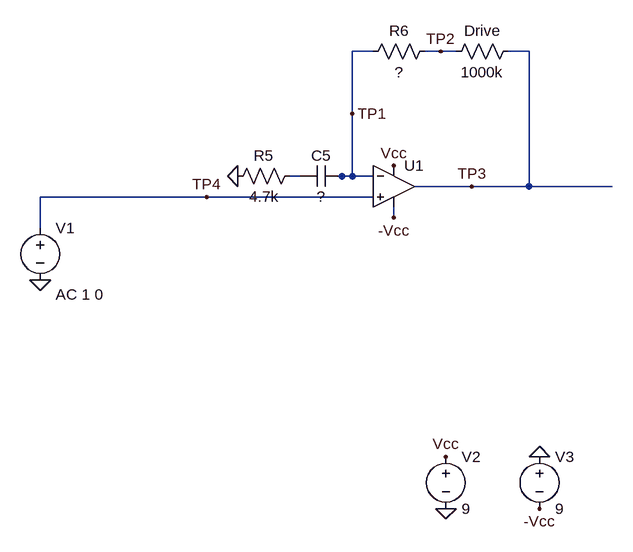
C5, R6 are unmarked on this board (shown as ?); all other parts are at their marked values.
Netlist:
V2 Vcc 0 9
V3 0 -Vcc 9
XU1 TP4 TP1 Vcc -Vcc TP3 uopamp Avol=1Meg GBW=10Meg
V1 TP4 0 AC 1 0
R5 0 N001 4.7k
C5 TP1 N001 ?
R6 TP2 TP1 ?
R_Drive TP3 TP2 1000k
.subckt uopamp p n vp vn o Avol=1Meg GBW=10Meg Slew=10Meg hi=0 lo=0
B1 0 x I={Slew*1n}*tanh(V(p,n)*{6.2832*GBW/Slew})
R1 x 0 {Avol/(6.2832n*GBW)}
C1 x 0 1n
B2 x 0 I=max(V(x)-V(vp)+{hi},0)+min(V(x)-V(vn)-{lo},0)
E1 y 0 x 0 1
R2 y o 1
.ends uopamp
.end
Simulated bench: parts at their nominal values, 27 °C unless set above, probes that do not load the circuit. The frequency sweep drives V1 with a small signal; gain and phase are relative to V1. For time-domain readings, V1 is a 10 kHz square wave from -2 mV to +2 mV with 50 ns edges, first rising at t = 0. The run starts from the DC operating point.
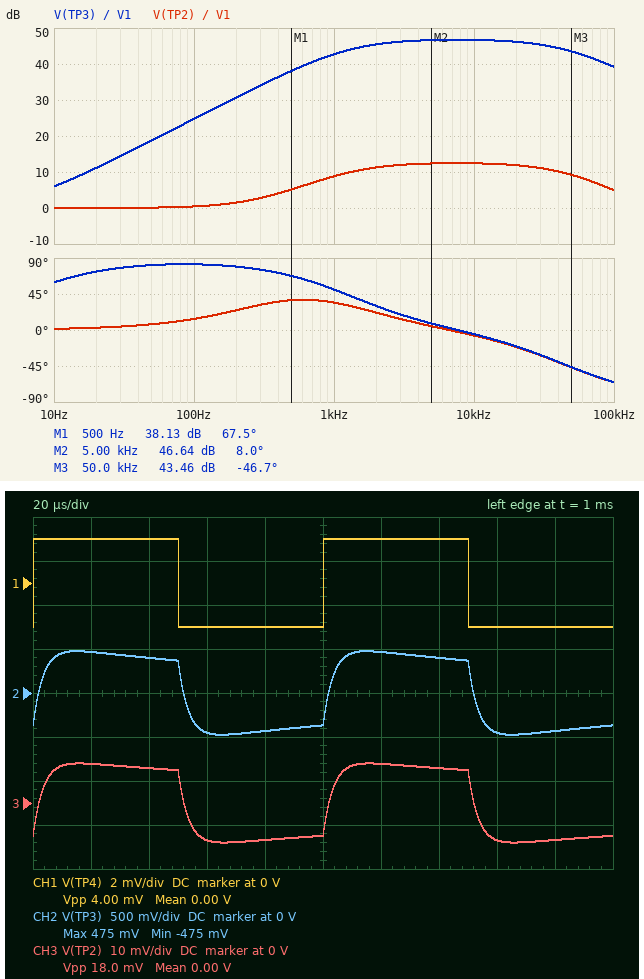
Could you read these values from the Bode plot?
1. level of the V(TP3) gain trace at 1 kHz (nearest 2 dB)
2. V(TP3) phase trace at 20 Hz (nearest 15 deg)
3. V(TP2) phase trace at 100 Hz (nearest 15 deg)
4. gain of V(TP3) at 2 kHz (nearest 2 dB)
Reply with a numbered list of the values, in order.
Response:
1. 42 dB
2. 75 deg
3. 15 deg
4. 46 dB
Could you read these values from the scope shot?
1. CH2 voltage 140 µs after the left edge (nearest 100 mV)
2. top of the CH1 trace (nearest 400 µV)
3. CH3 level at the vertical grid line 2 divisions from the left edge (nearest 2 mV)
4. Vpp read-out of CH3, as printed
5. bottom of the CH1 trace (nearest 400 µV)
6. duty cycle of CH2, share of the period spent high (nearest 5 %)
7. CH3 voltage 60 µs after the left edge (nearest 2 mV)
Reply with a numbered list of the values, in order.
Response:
1. 400 mV
2. 2.0 mV
3. 8 mV
4. 18.0 mV
5. -2.0 mV
6. 50 %
7. -8 mV
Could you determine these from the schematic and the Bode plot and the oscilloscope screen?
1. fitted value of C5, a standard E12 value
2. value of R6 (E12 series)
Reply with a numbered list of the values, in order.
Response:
1. 27 nF
2. 15 kΩ
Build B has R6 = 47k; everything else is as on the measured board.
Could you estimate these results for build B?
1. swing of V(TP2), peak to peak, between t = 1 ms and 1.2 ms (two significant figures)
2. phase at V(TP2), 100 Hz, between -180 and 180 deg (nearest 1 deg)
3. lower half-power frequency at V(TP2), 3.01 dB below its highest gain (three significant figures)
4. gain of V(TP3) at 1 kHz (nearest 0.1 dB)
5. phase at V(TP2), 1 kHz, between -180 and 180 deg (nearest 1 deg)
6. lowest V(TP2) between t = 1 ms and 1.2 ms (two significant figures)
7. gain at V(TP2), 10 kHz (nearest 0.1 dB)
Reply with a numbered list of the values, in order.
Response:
1. 48 mV
2. 37 deg
3. 1.21 kHz
4. 43.0 dB
5. 44 deg
6. -24 mV
7. 20.8 dB
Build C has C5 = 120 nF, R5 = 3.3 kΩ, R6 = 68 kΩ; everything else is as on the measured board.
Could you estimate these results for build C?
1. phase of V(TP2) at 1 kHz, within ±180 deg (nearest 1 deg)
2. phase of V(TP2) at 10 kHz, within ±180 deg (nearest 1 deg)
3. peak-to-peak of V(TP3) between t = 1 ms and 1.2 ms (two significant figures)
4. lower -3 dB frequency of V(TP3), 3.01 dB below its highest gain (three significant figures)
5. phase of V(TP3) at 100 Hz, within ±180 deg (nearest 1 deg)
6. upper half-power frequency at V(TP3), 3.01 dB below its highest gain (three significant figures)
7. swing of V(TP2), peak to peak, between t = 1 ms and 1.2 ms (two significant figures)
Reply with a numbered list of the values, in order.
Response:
1. 19 deg
2. -16 deg
3. 1.3 V
4. 397 Hz
5. 75 deg
6. 31.2 kHz
7. 88 mV
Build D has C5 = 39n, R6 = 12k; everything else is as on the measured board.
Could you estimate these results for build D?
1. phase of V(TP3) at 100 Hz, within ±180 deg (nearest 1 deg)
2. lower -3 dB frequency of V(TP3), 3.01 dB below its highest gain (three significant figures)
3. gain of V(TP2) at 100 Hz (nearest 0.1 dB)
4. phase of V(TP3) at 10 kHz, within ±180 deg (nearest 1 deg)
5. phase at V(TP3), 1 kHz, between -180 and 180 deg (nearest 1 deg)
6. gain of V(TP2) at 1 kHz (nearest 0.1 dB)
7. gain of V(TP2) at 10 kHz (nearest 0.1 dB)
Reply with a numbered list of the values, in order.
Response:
1. 81 deg
2. 852 Hz
3. 0.6 dB
4. -7 deg
5. 40 deg
6. 8.9 dB
7. 10.9 dB
